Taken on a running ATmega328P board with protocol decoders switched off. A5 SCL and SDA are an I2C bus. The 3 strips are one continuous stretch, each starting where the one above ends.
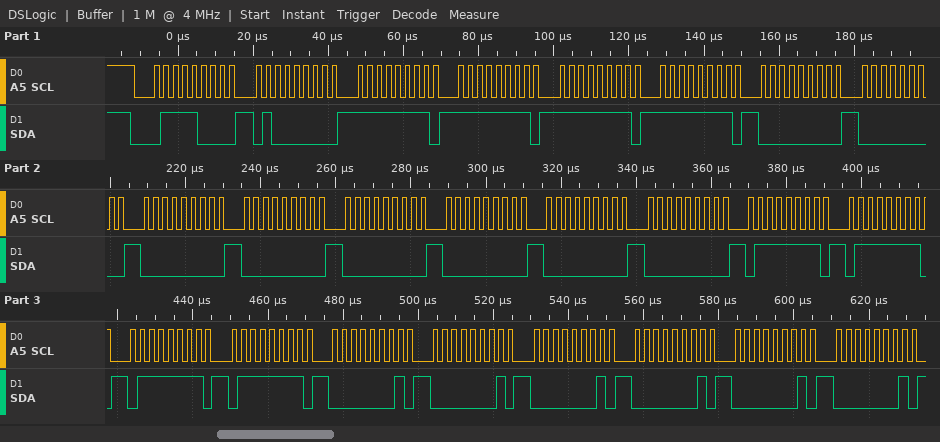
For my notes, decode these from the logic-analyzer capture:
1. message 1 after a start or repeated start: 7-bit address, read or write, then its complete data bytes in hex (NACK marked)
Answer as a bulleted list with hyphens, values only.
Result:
- 0x3C write: 40 FF FF FF FF 00 00 00 00 00 00 00 00 7F 7F 7F 7F 01 01 01 01 01 01
